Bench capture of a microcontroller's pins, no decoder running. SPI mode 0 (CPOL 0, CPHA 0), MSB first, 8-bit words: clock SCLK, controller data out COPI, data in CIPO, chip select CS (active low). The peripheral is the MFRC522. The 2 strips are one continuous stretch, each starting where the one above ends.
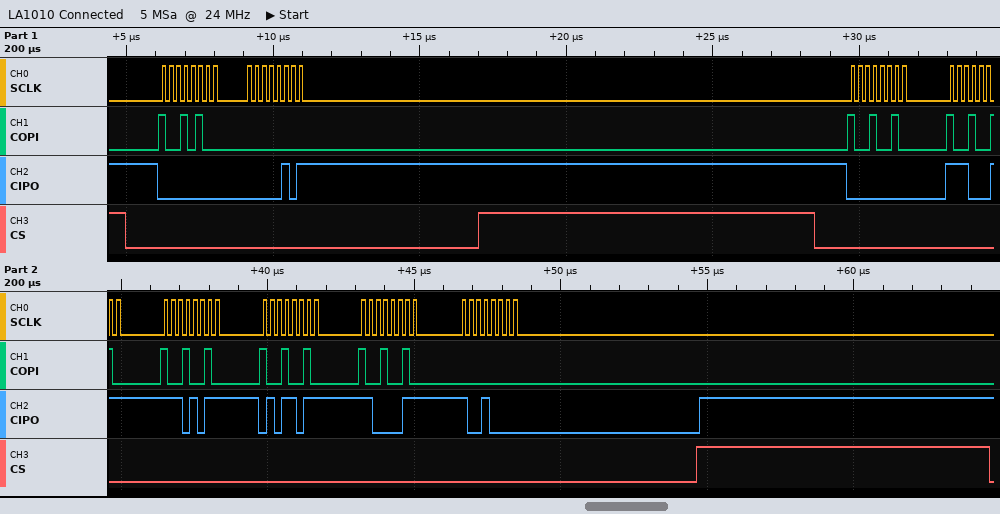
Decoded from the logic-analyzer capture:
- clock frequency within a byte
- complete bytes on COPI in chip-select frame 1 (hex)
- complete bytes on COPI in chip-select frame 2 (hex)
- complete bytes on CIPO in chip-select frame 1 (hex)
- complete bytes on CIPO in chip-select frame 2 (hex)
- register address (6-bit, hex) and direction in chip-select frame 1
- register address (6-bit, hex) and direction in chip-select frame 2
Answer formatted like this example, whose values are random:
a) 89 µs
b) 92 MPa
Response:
a) 4 MHz
b) 94 00
c) 92 92 92 92 92 00
d) 00 05
e) 00 E3 EB 5B C3 90
f) 0x0A read
g) 0x09 read
